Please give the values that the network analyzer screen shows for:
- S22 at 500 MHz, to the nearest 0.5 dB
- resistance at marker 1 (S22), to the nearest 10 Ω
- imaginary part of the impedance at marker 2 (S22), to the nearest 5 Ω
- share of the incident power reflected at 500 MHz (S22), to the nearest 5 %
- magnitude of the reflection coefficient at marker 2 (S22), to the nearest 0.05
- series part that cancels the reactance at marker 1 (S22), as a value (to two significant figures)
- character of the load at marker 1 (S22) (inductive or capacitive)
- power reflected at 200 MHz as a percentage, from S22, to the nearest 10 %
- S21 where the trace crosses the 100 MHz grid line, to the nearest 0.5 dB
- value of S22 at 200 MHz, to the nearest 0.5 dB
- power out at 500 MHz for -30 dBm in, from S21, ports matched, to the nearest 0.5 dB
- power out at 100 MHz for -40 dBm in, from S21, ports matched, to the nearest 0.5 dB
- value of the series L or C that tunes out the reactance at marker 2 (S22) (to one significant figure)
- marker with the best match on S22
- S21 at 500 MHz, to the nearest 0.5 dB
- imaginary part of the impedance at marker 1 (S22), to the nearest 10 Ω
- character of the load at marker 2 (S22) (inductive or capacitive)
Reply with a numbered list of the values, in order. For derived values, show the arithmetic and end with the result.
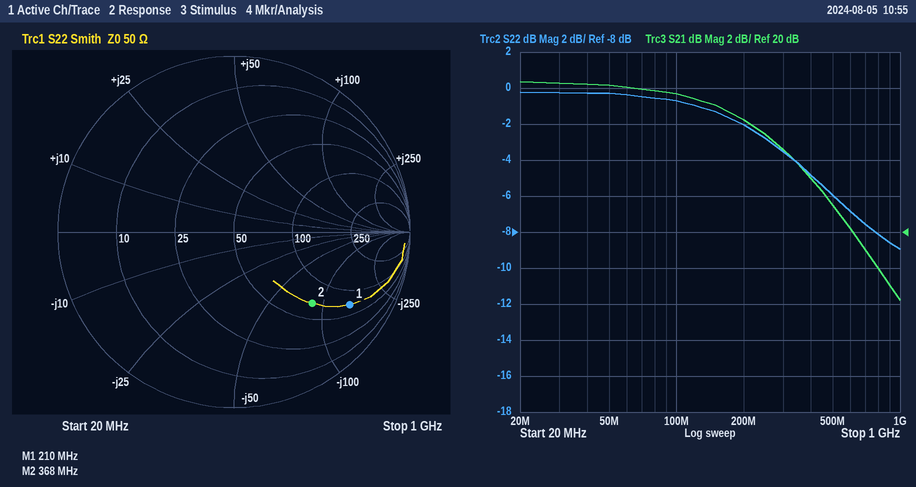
1. -6.0 dB
2. 70 Ω
3. -85 Ω
4. 10^(-6/10) ≈ 25 %
5. 0.60
6. L = 140 Ω/(2π × 210 MHz) ≈ 106 nH, so 110 nH to two significant figures
7. capacitive
8. 10^(-2/10) ≈ 63.1 %, so 60 % to the nearest 10 %
9. 27.5 dB
10. -2.0 dB
11. -30 dBm + (21.5 dB) = -8.5 dBm
12. -40 dBm + (27.5 dB) = -12.5 dBm
13. L = 85 Ω/(2π × 368 MHz) ≈ 36.8 nH, so 40 nH to one significant figure
14. marker 2
15. 21.5 dB
16. -140 Ω
17. capacitive
